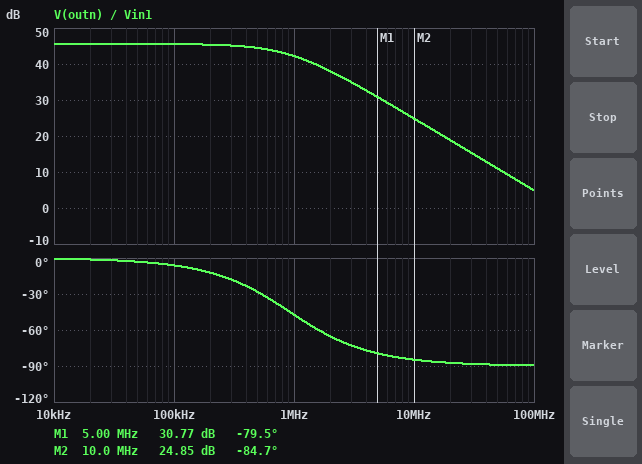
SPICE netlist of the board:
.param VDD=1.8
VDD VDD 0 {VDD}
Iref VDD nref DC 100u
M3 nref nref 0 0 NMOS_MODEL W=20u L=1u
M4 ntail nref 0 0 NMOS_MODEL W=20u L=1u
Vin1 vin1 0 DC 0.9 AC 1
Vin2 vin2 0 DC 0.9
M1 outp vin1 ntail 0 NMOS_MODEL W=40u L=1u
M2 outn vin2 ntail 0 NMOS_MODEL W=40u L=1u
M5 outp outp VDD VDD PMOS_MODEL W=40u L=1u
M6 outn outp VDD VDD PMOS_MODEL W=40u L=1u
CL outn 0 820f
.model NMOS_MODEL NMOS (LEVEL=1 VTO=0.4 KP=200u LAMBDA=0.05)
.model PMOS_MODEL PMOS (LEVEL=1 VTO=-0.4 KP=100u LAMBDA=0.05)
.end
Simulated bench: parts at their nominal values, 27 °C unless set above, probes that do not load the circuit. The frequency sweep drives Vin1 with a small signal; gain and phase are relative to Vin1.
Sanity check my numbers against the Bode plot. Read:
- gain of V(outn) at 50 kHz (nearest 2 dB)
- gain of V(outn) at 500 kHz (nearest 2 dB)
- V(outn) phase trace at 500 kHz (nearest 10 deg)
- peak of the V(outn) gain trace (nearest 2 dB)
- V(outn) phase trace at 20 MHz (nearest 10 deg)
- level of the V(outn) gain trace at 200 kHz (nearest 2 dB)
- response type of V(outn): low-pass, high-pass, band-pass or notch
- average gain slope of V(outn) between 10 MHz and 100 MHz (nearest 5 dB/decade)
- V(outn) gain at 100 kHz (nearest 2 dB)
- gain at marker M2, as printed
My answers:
46 dB
44 dB
-30 deg
46 dB
-90 deg
46 dB
low-pass
-20 dB/decade
46 dB
24.85 dB
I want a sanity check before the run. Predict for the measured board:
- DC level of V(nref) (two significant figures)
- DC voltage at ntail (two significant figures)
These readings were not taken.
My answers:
620 mV
390 mV
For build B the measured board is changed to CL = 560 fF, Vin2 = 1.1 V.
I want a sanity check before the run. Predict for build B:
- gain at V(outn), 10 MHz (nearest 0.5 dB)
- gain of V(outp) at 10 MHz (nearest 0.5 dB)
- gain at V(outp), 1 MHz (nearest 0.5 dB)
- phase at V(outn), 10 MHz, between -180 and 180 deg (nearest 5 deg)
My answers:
0.5 dB
-30.5 dB
-44.0 dB
0 deg
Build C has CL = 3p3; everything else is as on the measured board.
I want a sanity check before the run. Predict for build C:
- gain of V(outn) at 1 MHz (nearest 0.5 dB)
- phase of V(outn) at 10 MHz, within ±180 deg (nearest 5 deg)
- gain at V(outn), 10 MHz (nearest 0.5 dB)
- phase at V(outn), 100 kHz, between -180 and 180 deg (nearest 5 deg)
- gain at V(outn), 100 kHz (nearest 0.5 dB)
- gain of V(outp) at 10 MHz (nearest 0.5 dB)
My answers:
32.5 dB
-90 deg
13.0 dB
-25 deg
45.0 dB
-3.0 dB
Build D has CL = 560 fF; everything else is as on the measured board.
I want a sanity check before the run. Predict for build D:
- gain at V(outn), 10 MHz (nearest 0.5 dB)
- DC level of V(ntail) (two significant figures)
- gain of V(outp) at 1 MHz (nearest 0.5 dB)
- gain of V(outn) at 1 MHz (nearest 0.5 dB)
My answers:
28.0 dB
390 mV
-6.0 dB
43.5 dB
